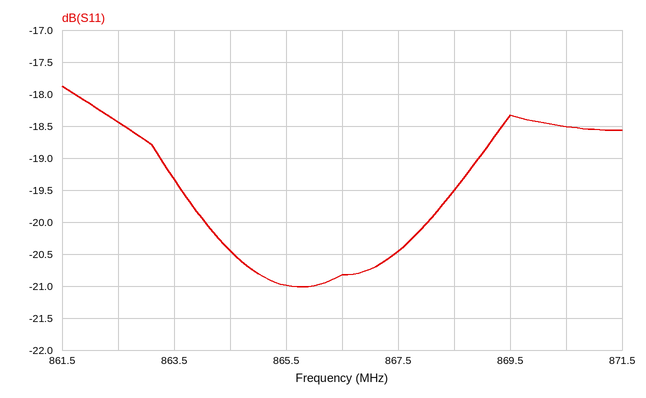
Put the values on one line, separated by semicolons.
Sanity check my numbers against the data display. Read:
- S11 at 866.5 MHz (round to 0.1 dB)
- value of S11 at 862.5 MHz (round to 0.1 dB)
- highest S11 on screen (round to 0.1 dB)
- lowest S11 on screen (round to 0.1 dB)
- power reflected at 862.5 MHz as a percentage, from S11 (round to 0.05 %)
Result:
-20.8 dB; -18.4 dB; -17.9 dB; -21.0 dB; 1.45 %
